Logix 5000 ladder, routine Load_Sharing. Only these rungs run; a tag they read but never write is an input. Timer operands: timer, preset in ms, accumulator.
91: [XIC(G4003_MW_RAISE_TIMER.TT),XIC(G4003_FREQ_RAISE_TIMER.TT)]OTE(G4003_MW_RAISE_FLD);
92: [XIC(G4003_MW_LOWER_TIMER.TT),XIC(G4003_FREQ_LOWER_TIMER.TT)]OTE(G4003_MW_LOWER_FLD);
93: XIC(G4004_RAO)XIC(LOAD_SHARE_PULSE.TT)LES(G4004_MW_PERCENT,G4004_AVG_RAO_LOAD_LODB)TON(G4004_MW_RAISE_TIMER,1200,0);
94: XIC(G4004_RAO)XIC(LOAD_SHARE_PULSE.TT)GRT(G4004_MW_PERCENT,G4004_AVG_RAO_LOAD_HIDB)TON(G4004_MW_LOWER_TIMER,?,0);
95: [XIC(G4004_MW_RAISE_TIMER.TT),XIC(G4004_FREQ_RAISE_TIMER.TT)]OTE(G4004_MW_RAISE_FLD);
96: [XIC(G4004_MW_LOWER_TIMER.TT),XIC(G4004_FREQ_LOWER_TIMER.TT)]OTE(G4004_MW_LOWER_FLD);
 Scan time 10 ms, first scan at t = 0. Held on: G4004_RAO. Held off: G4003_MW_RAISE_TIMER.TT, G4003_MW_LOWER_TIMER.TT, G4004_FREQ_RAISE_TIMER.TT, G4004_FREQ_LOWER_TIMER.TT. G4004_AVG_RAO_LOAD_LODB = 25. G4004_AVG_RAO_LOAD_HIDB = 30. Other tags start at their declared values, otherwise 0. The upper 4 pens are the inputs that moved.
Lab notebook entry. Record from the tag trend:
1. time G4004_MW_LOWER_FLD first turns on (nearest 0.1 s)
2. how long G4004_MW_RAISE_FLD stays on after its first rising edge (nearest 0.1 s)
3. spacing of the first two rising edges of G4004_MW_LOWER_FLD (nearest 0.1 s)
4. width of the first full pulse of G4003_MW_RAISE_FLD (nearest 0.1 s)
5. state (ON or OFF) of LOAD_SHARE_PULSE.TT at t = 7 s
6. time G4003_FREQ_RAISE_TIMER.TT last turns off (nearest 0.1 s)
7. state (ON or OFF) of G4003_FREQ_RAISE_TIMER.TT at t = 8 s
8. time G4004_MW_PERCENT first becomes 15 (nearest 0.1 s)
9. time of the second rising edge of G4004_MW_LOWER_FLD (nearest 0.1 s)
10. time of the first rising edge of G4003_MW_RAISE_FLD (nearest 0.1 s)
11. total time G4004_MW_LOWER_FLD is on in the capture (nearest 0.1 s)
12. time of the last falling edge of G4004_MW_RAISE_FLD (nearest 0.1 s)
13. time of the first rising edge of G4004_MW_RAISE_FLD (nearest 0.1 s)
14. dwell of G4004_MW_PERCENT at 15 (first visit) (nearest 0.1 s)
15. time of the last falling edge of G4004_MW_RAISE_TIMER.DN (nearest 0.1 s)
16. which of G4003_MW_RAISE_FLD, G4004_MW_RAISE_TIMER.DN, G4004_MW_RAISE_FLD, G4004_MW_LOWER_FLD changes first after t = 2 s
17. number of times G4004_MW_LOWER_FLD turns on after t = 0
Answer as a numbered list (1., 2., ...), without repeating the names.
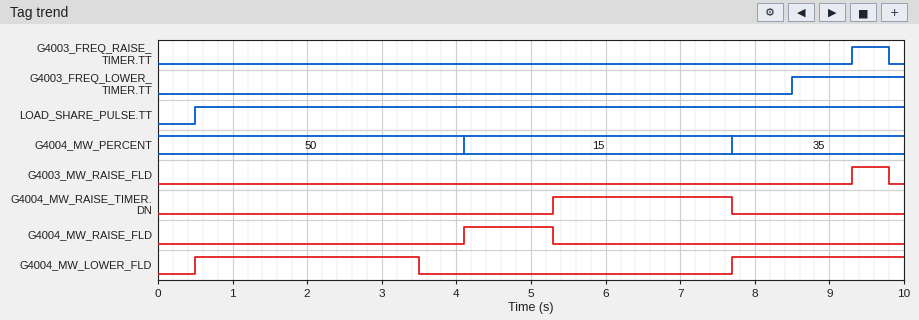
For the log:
1. 0.5 s
2. 1.2 s
3. 7.2 s
4. 0.5 s
5. ON
6. 9.8 s
7. OFF
8. 4.1 s
9. 7.7 s
10. 9.3 s
11. 5.3 s
12. 5.3 s
13. 4.1 s
14. 3.6 s
15. 7.7 s
16. G4004_MW_LOWER_FLD
17. 2
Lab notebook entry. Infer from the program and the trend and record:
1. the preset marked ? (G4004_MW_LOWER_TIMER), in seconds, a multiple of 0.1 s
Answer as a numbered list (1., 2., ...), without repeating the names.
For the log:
1. 3.0 s
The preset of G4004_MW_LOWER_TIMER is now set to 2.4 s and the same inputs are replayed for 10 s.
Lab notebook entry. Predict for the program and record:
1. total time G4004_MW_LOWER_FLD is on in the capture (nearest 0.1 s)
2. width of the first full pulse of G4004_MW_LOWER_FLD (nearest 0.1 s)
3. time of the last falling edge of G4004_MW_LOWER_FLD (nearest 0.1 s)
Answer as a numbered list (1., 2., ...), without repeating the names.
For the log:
1. 4.7 s
2. 2.4 s
3. 2.9 s
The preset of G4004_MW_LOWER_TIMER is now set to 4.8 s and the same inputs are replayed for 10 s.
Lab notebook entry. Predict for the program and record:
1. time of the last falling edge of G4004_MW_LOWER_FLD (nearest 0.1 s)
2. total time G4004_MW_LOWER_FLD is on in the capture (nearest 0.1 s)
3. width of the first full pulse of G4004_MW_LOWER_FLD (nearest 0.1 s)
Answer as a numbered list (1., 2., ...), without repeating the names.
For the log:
1. 4.1 s
2. 5.9 s
3. 3.6 s
